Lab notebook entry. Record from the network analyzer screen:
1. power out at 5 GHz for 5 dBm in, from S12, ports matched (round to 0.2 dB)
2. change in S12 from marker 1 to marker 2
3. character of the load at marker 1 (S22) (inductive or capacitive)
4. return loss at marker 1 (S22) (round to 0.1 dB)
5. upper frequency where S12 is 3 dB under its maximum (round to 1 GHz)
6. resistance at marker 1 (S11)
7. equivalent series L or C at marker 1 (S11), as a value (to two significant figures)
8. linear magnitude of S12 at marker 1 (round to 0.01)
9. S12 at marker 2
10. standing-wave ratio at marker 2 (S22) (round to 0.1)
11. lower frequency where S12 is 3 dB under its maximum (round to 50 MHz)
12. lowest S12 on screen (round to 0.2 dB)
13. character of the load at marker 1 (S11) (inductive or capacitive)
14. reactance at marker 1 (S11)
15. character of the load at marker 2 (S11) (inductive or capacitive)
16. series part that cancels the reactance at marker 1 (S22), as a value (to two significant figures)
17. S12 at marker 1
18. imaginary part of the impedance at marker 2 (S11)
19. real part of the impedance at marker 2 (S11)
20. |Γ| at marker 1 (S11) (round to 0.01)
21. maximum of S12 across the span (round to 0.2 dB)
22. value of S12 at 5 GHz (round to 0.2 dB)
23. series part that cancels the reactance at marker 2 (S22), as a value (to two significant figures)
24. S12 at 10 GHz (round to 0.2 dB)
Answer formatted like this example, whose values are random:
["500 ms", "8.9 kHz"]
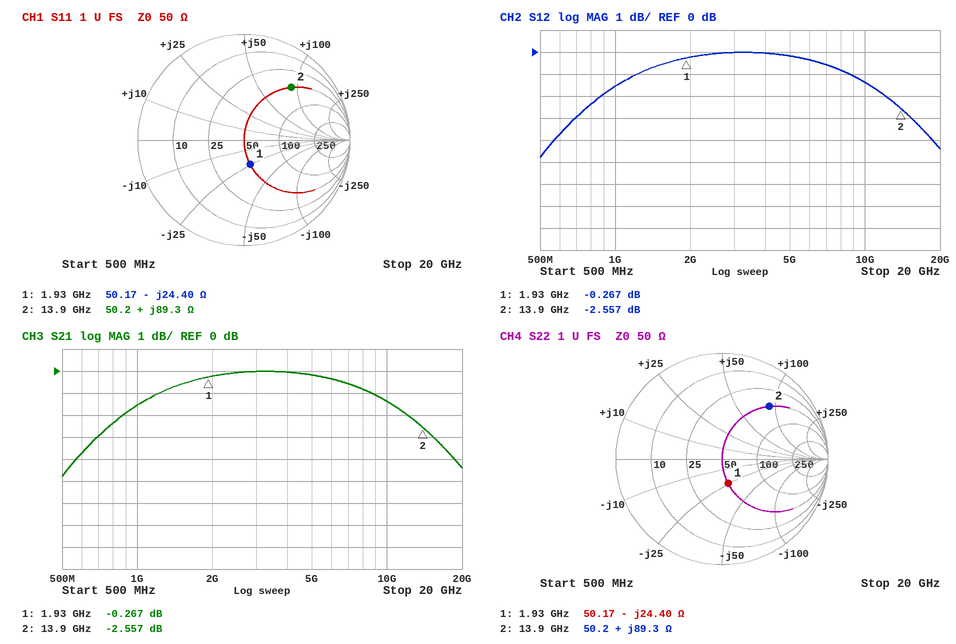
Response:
["4.8 dBm", "-2.290 dB", "capacitive", "12.5 dB", "15 GHz", "50.17 Ω", "3.4 pF", "0.97", "-2.557 dB", "5.0", "700 MHz", "-4.8 dB", "capacitive", "-24.40 Ω", "inductive", "2.0 nH", "-0.267 dB", "+89.3 Ω", "50.2 Ω", "0.24", "0.0 dB", "-0.2 dB", "130 fF", "-1.4 dB"]
